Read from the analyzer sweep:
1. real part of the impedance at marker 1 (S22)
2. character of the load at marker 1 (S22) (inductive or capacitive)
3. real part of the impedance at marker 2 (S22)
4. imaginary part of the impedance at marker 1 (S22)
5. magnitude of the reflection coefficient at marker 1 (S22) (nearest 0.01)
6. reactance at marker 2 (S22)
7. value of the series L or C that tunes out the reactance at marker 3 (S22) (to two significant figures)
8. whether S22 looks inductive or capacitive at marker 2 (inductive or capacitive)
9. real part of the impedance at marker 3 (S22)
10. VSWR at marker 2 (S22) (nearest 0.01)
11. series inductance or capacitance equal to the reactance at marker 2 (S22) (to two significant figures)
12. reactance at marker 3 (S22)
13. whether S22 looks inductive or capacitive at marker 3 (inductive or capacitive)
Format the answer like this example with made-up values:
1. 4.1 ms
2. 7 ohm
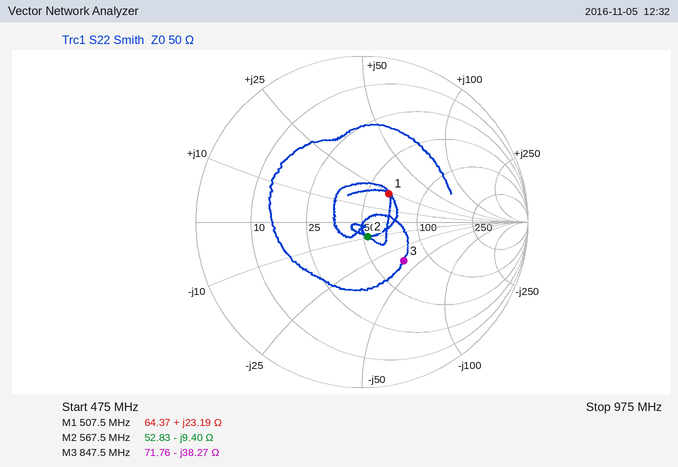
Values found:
1. 64.37 Ω
2. inductive
3. 52.83 Ω
4. +23.19 Ω
5. 0.23
6. -9.40 Ω
7. 7.2 nH
8. capacitive
9. 71.76 Ω
10. 1.21
11. 30 pF
12. -38.27 Ω
13. capacitive
